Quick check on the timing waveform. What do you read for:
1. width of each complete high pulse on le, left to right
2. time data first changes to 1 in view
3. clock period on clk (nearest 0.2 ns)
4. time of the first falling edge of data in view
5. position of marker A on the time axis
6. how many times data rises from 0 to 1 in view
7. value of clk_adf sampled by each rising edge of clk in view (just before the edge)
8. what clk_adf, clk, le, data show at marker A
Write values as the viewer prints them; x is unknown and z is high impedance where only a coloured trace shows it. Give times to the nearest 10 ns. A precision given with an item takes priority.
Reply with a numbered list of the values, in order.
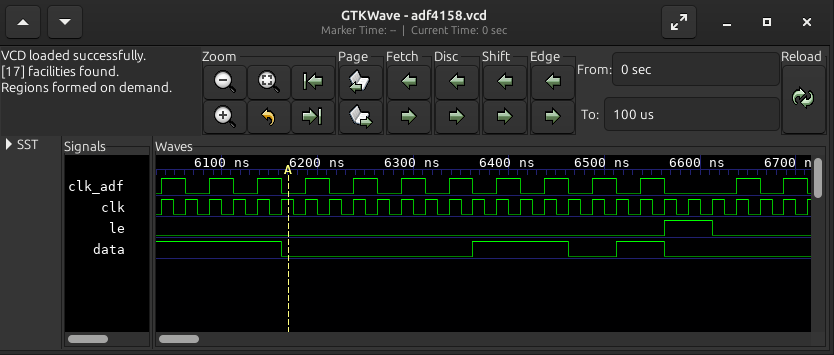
1. 50 ns
2. 6360 ns
3. 25 ns
4. 6160 ns
5. 6170 ns
6. 2
7. 0 1 0 1 0 1 0 1 0 1 0 1 0 1 0 1 0 1 0 1 0 1 0 0 0 1 0 1
8. clk_adf=0, clk=1, le=0, data=0
